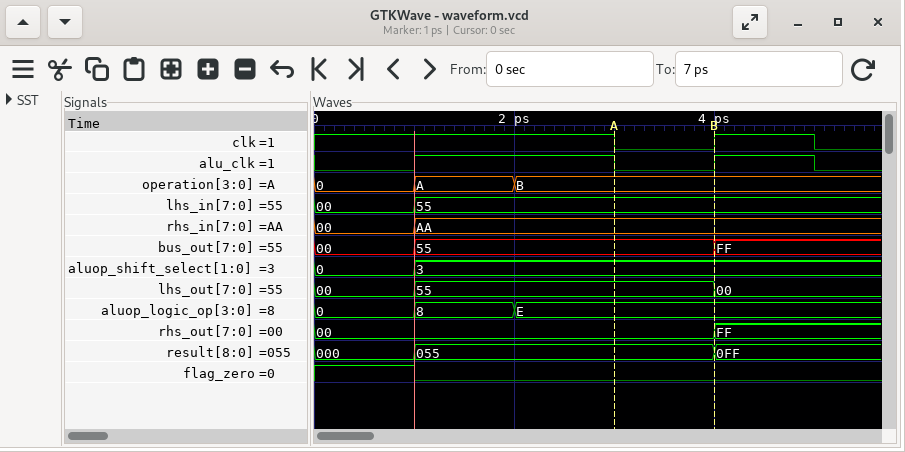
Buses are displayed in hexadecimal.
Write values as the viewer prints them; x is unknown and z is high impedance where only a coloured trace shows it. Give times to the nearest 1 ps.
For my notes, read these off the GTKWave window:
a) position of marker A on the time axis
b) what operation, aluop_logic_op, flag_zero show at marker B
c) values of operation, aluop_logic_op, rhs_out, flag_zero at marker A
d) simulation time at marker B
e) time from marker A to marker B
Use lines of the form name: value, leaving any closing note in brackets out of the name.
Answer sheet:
position of marker A on the time axis: 3 ps
what operation, aluop_logic_op, flag_zero show at marker B: operation=B, aluop_logic_op=E, flag_zero=0
values of operation, aluop_logic_op, rhs_out, flag_zero at marker A: operation=B, aluop_logic_op=E, rhs_out=00, flag_zero=0
simulation time at marker B: 4 ps
time from marker A to marker B: 1 ps
